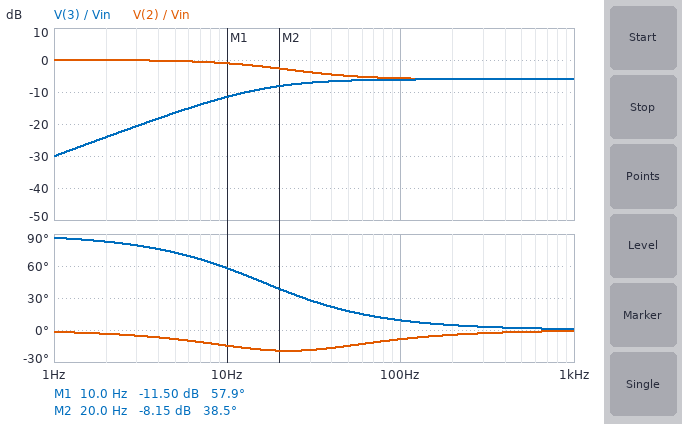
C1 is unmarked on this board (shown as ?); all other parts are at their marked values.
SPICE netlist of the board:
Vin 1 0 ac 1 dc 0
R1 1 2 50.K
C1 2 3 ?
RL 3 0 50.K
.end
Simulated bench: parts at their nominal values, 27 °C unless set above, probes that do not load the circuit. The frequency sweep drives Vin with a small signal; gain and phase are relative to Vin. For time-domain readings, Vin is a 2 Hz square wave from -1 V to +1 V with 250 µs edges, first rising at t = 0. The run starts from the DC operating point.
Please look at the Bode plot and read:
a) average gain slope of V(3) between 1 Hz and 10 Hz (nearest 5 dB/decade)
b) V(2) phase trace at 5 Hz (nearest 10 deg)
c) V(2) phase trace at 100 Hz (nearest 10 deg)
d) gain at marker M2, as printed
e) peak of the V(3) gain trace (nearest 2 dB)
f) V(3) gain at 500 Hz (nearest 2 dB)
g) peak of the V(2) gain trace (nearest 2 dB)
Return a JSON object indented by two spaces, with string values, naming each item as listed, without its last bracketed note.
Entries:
{
  "average gain slope of V(3) between 1 Hz and 10 Hz": "20 dB/decade",
  "V(2) phase trace at 5 Hz": "-10 deg",
  "V(2) phase trace at 100 Hz": "-10 deg",
  "gain at marker M2, as printed": "-8.15 dB",
  "peak of the V(3) gain trace": "-6 dB",
  "V(3) gain at 500 Hz": "-6 dB",
  "peak of the V(2) gain trace": "0 dB"
}
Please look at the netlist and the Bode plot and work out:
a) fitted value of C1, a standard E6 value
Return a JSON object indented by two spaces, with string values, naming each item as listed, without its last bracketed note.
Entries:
{
  "fitted value of C1, a standard E6 value": "100 nF"
}
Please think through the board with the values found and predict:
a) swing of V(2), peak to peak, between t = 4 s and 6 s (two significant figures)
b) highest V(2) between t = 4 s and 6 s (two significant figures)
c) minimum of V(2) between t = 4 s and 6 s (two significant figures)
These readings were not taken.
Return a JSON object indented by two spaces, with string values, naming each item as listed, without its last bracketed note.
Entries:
{
  "swing of V(2), peak to peak, between t = 4 s and 6 s": "2.0 V",
  "highest V(2) between t = 4 s and 6 s": "1.0 V",
  "minimum of V(2) between t = 4 s and 6 s": "-1.0 V"
}
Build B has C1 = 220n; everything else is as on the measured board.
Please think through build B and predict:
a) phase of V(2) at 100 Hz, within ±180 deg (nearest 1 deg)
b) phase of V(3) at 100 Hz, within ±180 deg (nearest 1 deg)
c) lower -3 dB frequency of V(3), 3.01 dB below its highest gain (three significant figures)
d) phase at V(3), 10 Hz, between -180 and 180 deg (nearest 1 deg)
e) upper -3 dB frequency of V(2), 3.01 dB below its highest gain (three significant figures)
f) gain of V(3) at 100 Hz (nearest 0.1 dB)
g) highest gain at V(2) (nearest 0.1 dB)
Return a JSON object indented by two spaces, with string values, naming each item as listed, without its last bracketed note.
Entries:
{
  "phase of V(2) at 100 Hz, within ±180 deg": "-4 deg",
  "phase of V(3) at 100 Hz, within ±180 deg": "4 deg",
  "lower -3 dB frequency of V(3), 3.01 dB below its highest gain": "7.23 Hz",
  "phase at V(3), 10 Hz, between -180 and 180 deg": "36 deg",
  "upper -3 dB frequency of V(2), 3.01 dB below its highest gain": "10.2 Hz",
  "gain of V(3) at 100 Hz": "-6.0 dB",
  "highest gain at V(2)": "0 dB"
}
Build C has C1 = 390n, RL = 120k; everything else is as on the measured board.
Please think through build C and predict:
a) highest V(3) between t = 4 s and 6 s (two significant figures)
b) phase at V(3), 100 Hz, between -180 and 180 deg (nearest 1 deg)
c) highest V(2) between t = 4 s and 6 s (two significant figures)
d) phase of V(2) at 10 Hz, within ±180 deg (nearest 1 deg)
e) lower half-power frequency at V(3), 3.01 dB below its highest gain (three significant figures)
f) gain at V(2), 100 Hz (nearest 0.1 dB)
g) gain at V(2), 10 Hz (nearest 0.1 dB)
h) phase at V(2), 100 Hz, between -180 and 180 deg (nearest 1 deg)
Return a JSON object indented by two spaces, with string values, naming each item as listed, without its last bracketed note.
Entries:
{
  "highest V(3) between t = 4 s and 6 s": "1.4 V",
  "phase at V(3), 100 Hz, between -180 and 180 deg": "1 deg",
  "highest V(2) between t = 4 s and 6 s": "990 mV",
  "phase of V(2) at 10 Hz, within ±180 deg": "-5 deg",
  "lower half-power frequency at V(3), 3.01 dB below its highest gain": "2.40 Hz",
  "gain at V(2), 100 Hz": "-3.0 dB",
  "gain at V(2), 10 Hz": "-2.8 dB",
  "phase at V(2), 100 Hz, between -180 and 180 deg": "-1 deg"
}
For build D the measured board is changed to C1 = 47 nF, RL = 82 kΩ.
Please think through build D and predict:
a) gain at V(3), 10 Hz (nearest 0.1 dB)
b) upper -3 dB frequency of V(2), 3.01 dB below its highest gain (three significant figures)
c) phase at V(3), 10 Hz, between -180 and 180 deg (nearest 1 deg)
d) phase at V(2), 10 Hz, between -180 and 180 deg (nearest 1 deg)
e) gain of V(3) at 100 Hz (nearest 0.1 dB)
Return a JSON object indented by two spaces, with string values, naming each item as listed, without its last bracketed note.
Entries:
{
  "gain at V(3), 10 Hz": "-12.9 dB",
  "upper -3 dB frequency of V(2), 3.01 dB below its highest gain": "53.7 Hz",
  "phase at V(3), 10 Hz, between -180 and 180 deg": "69 deg",
  "phase at V(2), 10 Hz, between -180 and 180 deg": "-8 deg",
  "gain of V(3) at 100 Hz": "-4.4 dB"
}
